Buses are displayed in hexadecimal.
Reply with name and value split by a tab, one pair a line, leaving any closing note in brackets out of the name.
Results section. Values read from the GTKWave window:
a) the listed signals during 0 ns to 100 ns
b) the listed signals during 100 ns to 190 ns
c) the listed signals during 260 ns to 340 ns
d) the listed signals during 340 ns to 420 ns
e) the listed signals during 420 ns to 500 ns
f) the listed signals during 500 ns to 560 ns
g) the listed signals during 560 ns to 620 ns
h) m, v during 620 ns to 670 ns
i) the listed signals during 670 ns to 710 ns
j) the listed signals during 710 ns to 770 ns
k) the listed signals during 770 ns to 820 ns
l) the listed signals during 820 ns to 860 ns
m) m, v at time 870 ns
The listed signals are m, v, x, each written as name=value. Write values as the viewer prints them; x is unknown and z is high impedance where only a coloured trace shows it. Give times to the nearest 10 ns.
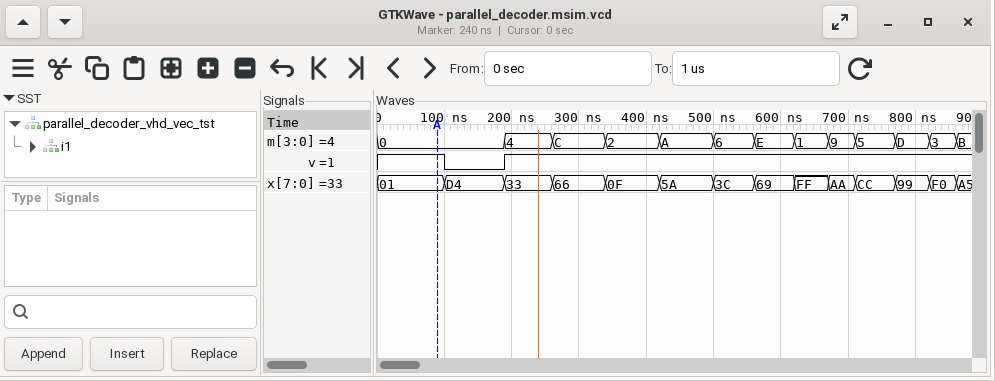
the listed signals during 0 ns to 100 ns	m=0, v=1, x=01
the listed signals during 100 ns to 190 ns	m=0, v=0, x=D4
the listed signals during 260 ns to 340 ns	m=C, v=1, x=66
the listed signals during 340 ns to 420 ns	m=2, v=1, x=0F
the listed signals during 420 ns to 500 ns	m=A, v=1, x=5A
the listed signals during 500 ns to 560 ns	m=6, v=1, x=3C
the listed signals during 560 ns to 620 ns	m=E, v=1, x=69
m, v during 620 ns to 670 ns	m=1, v=1
the listed signals during 670 ns to 710 ns	m=9, v=1, x=AA
the listed signals during 710 ns to 770 ns	m=5, v=1, x=CC
the listed signals during 770 ns to 820 ns	m=D, v=1, x=99
the listed signals during 820 ns to 860 ns	m=3, v=1, x=F0
m, v at time 870 ns	m=B, v=1
